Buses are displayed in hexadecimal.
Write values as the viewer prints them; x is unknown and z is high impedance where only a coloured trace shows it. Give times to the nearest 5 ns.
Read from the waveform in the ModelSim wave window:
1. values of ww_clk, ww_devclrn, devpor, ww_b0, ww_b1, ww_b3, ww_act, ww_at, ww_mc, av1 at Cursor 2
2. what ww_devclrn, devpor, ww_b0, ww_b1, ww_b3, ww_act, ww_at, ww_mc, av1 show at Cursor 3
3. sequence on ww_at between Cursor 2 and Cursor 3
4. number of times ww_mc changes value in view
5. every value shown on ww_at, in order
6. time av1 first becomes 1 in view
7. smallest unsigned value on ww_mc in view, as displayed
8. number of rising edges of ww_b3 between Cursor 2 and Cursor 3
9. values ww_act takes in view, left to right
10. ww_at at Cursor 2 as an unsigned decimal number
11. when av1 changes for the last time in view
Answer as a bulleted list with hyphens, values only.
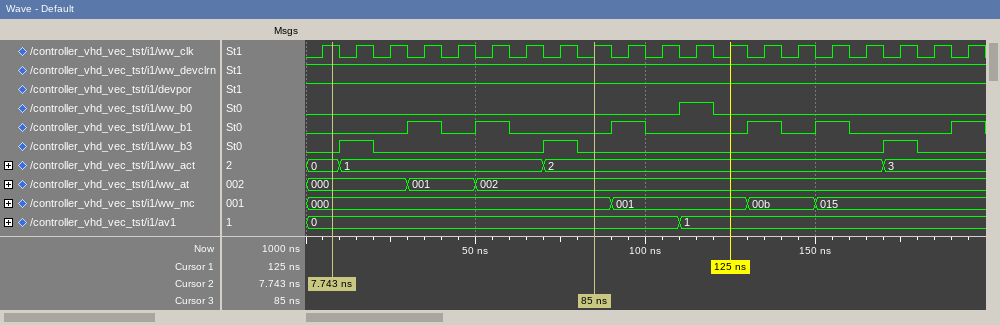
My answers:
- ww_clk=1, ww_devclrn=1, devpor=1, ww_b0=0, ww_b1=0, ww_b3=0, ww_act=0, ww_at=000, ww_mc=000, av1=0
- ww_devclrn=1, devpor=1, ww_b0=0, ww_b1=0, ww_b3=0, ww_act=2, ww_at=002, ww_mc=000, av1=0
- 000, 001, 002
- 3
- 000, 001, 002
- 110 ns
- 000
- 2
- 0, 1, 2, 3
- 0
- 110 ns
